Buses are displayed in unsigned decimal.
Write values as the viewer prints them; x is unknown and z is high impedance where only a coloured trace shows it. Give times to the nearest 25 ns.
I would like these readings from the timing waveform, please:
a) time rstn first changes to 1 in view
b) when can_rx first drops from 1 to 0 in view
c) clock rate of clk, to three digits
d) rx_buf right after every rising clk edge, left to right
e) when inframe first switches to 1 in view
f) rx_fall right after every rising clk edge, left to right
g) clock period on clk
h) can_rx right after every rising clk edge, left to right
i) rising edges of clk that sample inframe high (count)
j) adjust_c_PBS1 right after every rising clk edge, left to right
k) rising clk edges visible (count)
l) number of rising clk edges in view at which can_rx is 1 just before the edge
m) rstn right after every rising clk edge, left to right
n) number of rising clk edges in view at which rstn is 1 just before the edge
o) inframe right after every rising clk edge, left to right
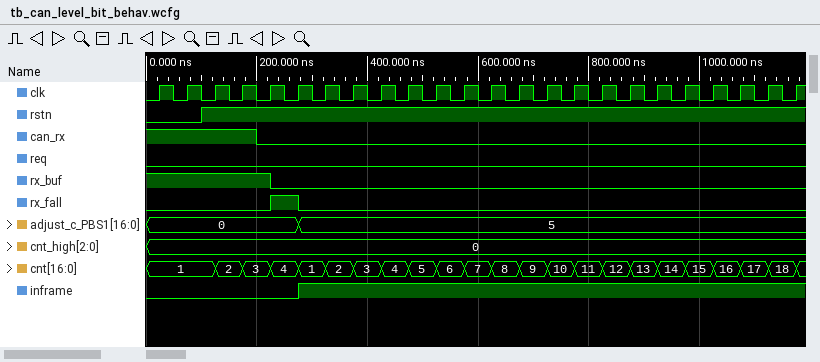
100 ns
200 ns
20.0 MHz
1 1 1 1 0 0 0 0 0 0 0 0 0 0 0 0 0 0 0 0 0 0 0 0
275 ns
0 0 0 0 1 0 0 0 0 0 0 0 0 0 0 0 0 0 0 0 0 0 0 0
50 ns
1 1 1 1 0 0 0 0 0 0 0 0 0 0 0 0 0 0 0 0 0 0 0 0
18
0, 0, 0, 0, 0, 5, 5, 5, 5, 5, 5, 5, 5, 5, 5, 5, 5, 5, 5, 5, 5, 5, 5, 5
24
4
0 0 1 1 1 1 1 1 1 1 1 1 1 1 1 1 1 1 1 1 1 1 1 1
22
0 0 0 0 0 1 1 1 1 1 1 1 1 1 1 1 1 1 1 1 1 1 1 1
